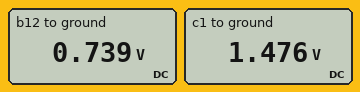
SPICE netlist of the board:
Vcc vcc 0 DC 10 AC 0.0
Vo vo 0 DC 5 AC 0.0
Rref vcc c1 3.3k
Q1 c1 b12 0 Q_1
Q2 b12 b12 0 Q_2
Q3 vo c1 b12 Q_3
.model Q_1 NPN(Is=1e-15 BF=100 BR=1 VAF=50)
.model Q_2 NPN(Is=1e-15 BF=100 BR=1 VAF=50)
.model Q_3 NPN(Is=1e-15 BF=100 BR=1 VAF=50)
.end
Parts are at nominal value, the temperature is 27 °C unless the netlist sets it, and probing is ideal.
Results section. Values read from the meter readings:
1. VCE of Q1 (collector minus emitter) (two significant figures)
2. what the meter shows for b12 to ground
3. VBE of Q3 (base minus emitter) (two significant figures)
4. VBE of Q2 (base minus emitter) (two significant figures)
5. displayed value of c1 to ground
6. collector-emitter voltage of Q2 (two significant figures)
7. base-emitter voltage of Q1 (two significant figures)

1.5 V
0.739 V
740 mV
740 mV
1.476 V
740 mV
740 mV
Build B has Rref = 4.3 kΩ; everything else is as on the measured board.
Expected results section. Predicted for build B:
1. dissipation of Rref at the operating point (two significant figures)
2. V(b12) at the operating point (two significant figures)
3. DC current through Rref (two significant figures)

17 mW
730 mV
2.0 mA
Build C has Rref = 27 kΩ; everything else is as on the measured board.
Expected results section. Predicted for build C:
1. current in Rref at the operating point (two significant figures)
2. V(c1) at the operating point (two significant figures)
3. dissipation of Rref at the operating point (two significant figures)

320 µA
1.4 V
2.8 mW
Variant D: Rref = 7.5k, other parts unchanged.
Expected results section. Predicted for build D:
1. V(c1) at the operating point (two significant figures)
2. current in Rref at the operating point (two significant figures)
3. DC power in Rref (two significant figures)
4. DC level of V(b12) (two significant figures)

1.4 V
1.1 mA
9.8 mW
720 mV
